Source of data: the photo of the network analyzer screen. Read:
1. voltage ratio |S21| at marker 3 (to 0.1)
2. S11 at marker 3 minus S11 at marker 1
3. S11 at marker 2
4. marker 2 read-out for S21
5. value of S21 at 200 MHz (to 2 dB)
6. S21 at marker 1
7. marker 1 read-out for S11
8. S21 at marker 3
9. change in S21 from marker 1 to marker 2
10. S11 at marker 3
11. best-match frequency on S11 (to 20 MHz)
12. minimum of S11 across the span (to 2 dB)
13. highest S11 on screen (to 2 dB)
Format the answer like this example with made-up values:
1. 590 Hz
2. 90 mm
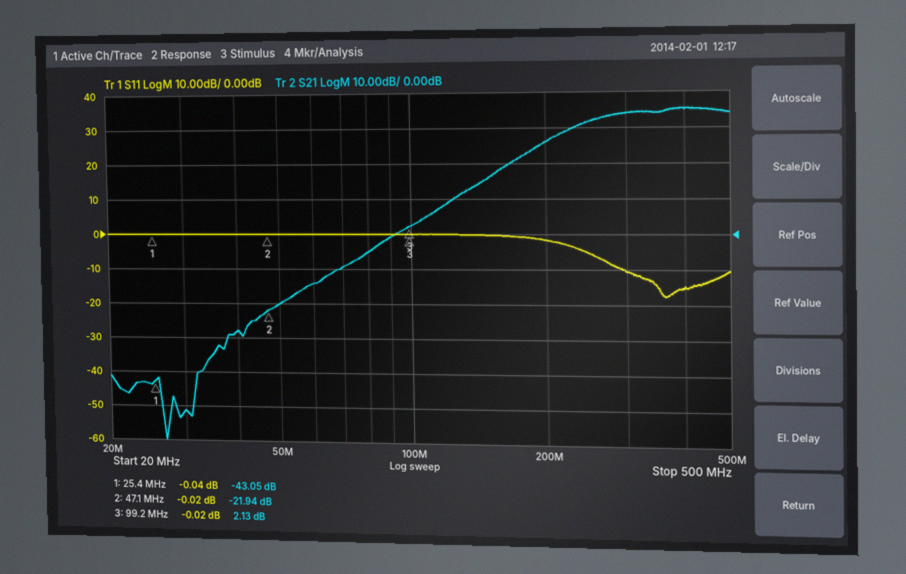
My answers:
1. 1.3
2. 0.02 dB
3. -0.02 dB
4. -21.94 dB
5. 26 dB
6. -43.05 dB
7. -0.04 dB
8. 2.13 dB
9. 21.11 dB
10. -0.02 dB
11. 360 MHz
12. -18 dB
13. 0 dB
